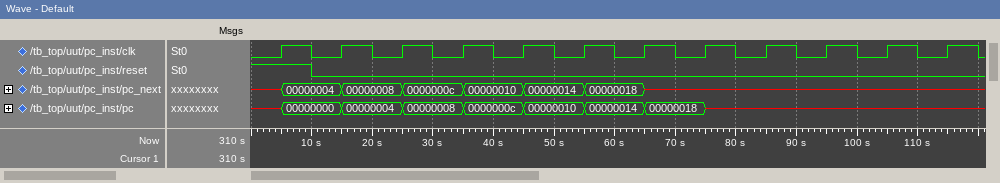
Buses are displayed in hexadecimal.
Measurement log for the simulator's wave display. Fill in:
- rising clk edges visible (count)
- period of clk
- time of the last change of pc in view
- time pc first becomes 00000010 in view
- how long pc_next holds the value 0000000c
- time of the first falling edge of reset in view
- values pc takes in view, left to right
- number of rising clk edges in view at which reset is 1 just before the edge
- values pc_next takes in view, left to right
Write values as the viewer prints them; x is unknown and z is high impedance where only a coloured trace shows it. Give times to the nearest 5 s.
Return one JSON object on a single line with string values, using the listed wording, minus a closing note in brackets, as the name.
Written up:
{"rising clk edges visible": "12", "period of clk": "10 s", "time of the last change of pc in view": "75 s", "time pc first becomes 00000010 in view": "45 s", "how long pc_next holds the value 0000000c": "10 s", "time of the first falling edge of reset in view": "10 s", "values pc takes in view, left to right": "x, 00000000, 00000004, 00000008, 0000000c, 00000010, 00000014, 00000018, x", "number of rising clk edges in view at which reset is 1 just before the edge": "1", "values pc_next takes in view, left to right": "x, 00000004, 00000008, 0000000c, 00000010, 00000014, 00000018, x"}
